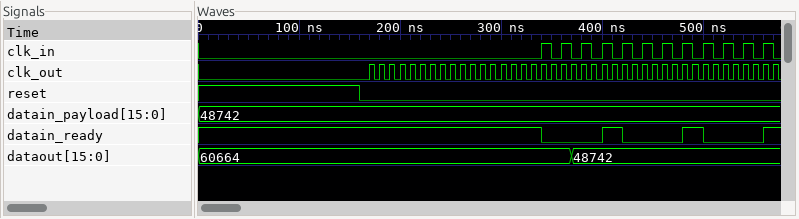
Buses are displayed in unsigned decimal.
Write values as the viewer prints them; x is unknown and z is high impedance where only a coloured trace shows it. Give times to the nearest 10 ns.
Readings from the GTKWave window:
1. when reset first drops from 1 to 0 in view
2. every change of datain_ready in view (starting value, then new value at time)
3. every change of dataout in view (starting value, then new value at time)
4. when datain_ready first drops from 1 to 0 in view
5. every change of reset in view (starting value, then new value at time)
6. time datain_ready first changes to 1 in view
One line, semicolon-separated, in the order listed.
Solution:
160 ns; 1, 0 at 340 ns, 1 at 400 ns, 0 at 420 ns, 1 at 480 ns, 0 at 500 ns, 1 at 560 ns; 60664, 48742 at 370 ns; 340 ns; 1, 0 at 160 ns; 400 ns
